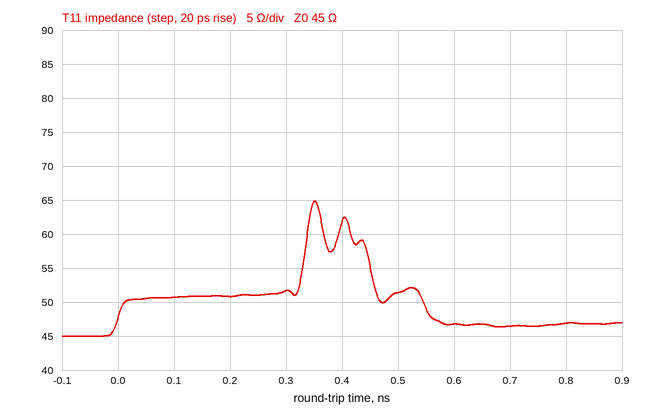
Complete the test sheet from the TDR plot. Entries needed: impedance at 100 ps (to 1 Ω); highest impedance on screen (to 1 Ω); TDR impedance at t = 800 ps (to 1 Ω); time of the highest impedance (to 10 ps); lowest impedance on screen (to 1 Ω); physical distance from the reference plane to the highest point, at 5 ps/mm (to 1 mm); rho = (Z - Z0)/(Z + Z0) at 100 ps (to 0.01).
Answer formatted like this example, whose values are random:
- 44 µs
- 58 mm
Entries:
- 51 Ω
- 65 Ω
- 47 Ω
- 350 ps
- 45 Ω
- 35 mm
- +0.06
